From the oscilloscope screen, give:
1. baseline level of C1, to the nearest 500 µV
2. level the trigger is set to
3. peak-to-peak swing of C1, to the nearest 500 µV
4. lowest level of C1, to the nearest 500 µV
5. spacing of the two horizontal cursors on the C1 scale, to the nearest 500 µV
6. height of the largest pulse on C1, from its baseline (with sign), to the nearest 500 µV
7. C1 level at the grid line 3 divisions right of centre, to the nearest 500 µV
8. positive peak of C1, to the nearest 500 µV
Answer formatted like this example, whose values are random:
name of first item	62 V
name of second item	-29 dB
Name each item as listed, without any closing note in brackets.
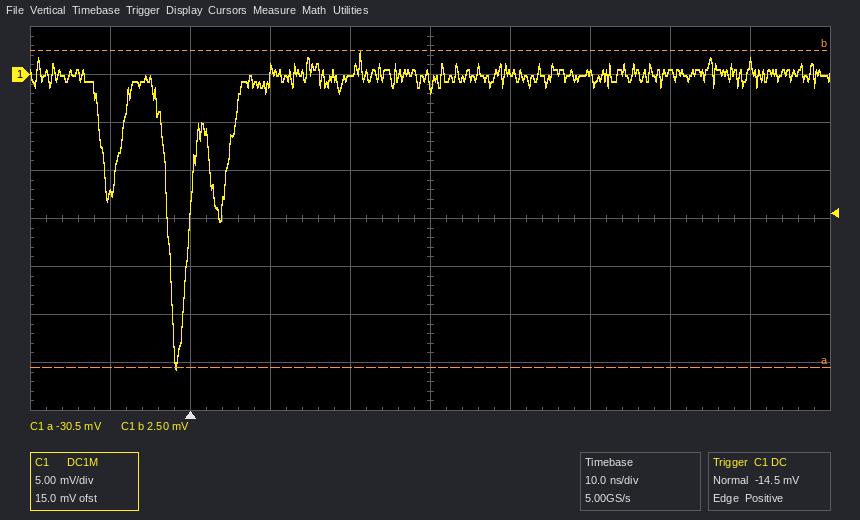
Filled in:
baseline level of C1, to the nearest 500 µV	0.0 mV
level the trigger is set to	-14.5 mV
peak-to-peak swing of C1, to the nearest 500 µV	33.0 mV
lowest level of C1, to the nearest 500 µV	-30.5 mV
spacing of the two horizontal cursors on the C1 scale, to the nearest 500 µV	33.0 mV
height of the largest pulse on C1, from its baseline (with sign), to the nearest 500 µV	-30.5 mV
C1 level at the grid line 3 divisions right of centre, to the nearest 500 µV	0.0 mV
positive peak of C1, to the nearest 500 µV	2.5 mV
